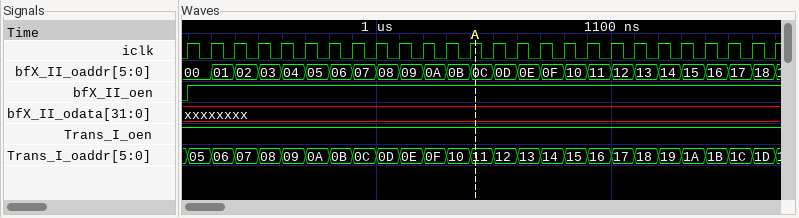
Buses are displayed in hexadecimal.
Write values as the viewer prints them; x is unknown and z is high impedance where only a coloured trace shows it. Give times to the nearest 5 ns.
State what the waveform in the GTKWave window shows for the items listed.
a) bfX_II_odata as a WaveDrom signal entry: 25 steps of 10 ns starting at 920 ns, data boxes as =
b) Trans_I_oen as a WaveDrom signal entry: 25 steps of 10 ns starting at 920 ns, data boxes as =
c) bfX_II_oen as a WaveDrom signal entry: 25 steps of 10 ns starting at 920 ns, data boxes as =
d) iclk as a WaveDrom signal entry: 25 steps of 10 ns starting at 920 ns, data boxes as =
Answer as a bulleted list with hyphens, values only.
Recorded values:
- {name: 'bfX_II_odata', wave: 'x........................'}
- {name: 'Trans_I_oen', wave: '1........................'}
- {name: 'bfX_II_oen', wave: '1........................'}
- {name: 'iclk', wave: 'p........................'}
